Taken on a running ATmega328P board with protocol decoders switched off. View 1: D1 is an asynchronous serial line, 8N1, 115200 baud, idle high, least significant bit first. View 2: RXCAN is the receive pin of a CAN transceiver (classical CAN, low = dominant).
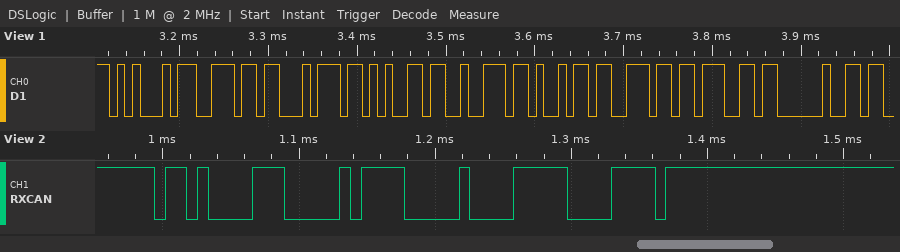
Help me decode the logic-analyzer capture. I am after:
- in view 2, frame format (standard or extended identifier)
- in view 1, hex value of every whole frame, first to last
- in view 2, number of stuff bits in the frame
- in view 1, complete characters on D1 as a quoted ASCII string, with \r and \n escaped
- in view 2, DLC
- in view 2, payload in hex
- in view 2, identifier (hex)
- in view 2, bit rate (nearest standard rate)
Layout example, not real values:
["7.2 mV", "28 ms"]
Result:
["standard", "45 6E 74 65 72 69 6E 67 20", "3", "\"Entering \"", "1", "E0", "0x687", "125 kbit/s"]
